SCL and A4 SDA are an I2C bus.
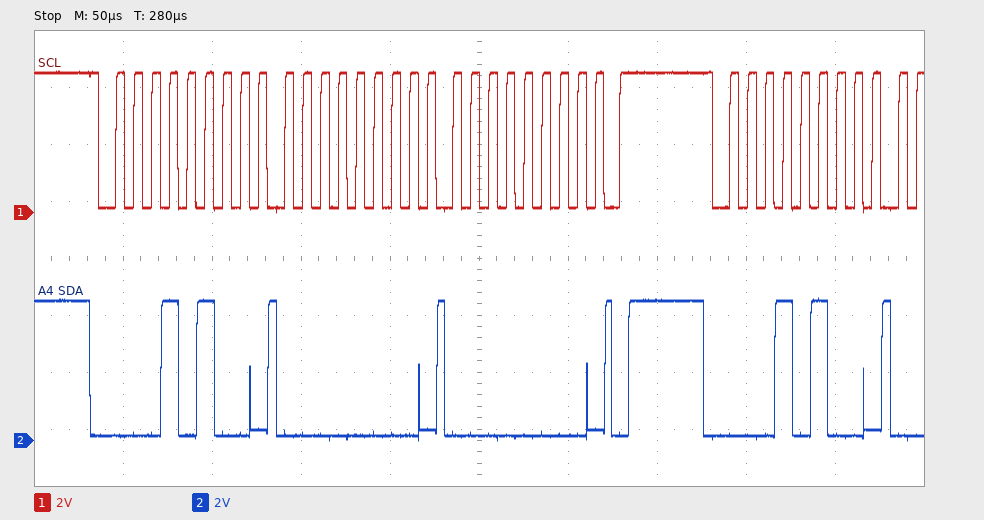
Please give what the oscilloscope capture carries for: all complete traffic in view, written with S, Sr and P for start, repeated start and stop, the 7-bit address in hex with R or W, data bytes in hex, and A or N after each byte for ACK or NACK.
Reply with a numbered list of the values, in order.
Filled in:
1. S 0AW A 00 A 00 A P S 0AW A
